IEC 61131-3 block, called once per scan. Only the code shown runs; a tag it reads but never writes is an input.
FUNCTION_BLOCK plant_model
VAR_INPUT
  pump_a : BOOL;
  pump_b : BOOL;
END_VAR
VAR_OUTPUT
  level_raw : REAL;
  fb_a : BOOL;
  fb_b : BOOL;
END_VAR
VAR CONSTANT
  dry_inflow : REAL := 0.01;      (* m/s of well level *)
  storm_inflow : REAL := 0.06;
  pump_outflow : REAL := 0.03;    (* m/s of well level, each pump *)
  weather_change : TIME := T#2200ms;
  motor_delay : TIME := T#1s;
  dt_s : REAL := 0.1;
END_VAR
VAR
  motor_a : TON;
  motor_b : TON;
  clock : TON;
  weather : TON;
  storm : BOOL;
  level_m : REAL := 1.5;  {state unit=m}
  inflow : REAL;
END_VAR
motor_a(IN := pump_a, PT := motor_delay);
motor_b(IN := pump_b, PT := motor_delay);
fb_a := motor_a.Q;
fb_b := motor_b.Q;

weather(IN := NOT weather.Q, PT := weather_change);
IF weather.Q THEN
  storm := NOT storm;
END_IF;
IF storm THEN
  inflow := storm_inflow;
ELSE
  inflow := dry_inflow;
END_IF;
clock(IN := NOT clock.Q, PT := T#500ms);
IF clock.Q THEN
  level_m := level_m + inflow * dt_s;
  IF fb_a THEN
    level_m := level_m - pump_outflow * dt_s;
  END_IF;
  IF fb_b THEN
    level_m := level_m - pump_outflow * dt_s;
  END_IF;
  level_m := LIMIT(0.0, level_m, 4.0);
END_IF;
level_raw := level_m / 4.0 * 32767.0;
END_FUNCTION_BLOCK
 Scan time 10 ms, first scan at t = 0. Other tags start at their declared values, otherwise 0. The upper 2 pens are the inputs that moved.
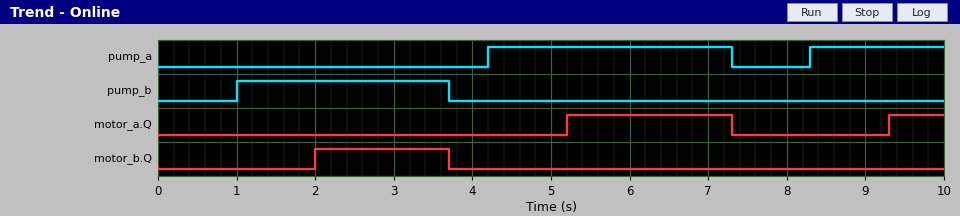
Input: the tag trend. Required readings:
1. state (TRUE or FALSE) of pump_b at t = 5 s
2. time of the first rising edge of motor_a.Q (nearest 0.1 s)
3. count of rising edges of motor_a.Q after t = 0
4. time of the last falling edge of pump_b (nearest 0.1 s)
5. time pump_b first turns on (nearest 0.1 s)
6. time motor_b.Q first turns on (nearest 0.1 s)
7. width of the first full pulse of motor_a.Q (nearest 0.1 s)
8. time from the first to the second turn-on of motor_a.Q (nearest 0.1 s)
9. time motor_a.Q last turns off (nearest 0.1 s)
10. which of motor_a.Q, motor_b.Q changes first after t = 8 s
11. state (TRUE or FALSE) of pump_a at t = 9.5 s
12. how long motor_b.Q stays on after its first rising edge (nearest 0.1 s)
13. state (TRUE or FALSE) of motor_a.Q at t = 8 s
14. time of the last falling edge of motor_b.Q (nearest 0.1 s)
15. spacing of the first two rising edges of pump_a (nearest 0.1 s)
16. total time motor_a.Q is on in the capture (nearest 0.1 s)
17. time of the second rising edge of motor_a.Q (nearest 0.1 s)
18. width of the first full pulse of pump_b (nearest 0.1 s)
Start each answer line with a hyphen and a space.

- FALSE
- 5.2 s
- 2
- 3.7 s
- 1.0 s
- 2.0 s
- 2.1 s
- 4.1 s
- 7.3 s
- motor_a.Q
- TRUE
- 1.7 s
- FALSE
- 3.7 s
- 4.1 s
- 2.8 s
- 9.3 s
- 2.7 s
